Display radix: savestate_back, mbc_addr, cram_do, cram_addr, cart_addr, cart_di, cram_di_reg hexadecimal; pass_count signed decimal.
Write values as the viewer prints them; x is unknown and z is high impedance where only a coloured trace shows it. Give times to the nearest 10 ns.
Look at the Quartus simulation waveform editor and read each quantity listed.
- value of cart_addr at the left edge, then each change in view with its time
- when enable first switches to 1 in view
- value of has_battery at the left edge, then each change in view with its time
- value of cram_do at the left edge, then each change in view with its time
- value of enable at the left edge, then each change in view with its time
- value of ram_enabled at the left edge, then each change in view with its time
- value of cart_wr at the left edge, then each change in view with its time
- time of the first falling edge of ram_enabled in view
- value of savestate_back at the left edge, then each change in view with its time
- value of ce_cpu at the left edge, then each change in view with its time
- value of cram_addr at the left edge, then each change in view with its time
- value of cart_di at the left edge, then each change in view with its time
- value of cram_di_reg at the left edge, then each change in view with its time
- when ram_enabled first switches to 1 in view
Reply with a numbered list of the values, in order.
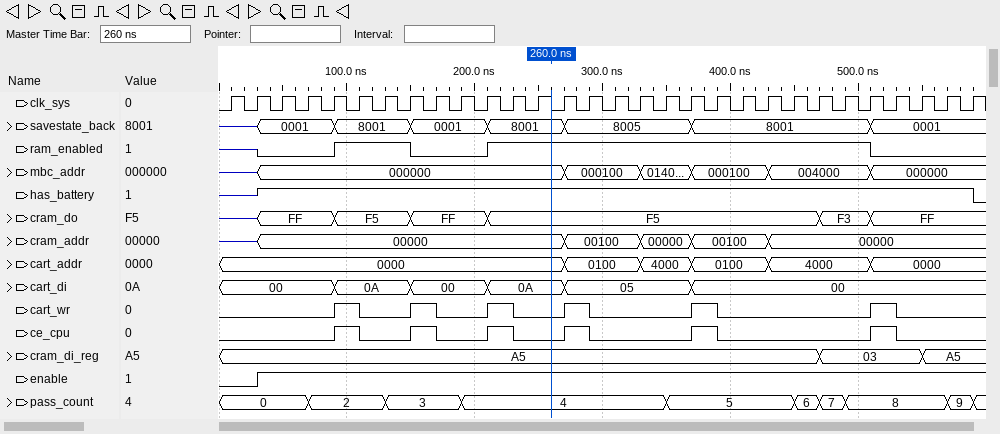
1. 0000, 0100 at 270 ns, 4000 at 330 ns, 0100 at 370 ns, 4000 at 430 ns, 0000 at 510 ns
2. 30 ns
3. z, 1 at 30 ns, 0 at 590 ns
4. z, FF at 30 ns, F5 at 90 ns, FF at 150 ns, F5 at 210 ns, F3 at 470 ns, FF at 510 ns
5. 0, 1 at 30 ns
6. z, 0 at 30 ns, 1 at 90 ns, 0 at 150 ns, 1 at 210 ns, 0 at 510 ns
7. 0, 1 at 90 ns, 0 at 110 ns, 1 at 150 ns, 0 at 170 ns, 1 at 210 ns, 0 at 230 ns, 1 at 270 ns, 0 at 290 ns, 1 at 370 ns, 0 at 390 ns, 1 at 510 ns, 0 at 530 ns
8. 150 ns
9. z, 0001 at 30 ns, 8001 at 90 ns, 0001 at 150 ns, 8001 at 210 ns, 8005 at 270 ns, 8001 at 370 ns, 0001 at 510 ns
10. 0, 1 at 90 ns, 0 at 110 ns, 1 at 150 ns, 0 at 170 ns, 1 at 210 ns, 0 at 230 ns, 1 at 270 ns, 0 at 290 ns, 1 at 370 ns, 0 at 390 ns, 1 at 510 ns, 0 at 530 ns
11. z, 00000 at 30 ns, 00100 at 270 ns, 00000 at 330 ns, 00100 at 370 ns, 00000 at 430 ns
12. 00, 0A at 90 ns, 00 at 150 ns, 0A at 210 ns, 05 at 270 ns, 00 at 370 ns
13. A5, 03 at 470 ns, A5 at 550 ns
14. 90 ns
